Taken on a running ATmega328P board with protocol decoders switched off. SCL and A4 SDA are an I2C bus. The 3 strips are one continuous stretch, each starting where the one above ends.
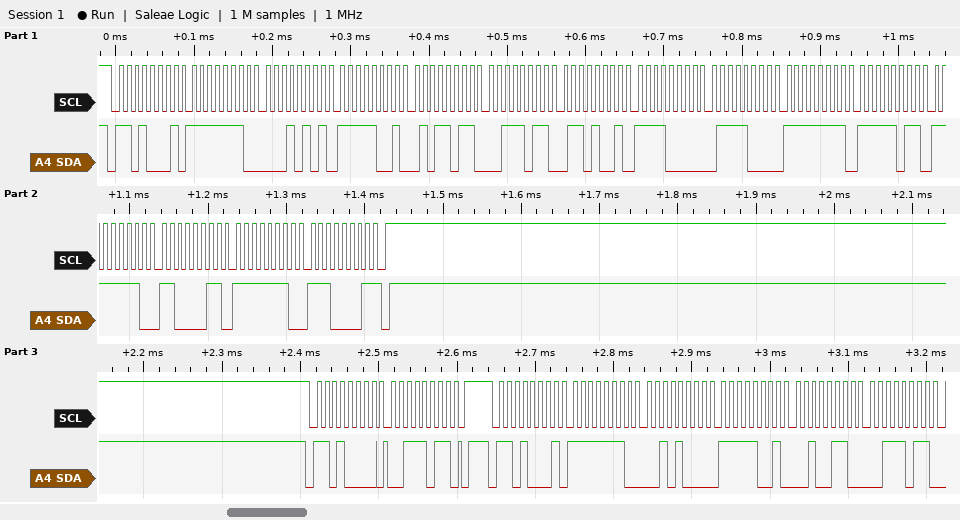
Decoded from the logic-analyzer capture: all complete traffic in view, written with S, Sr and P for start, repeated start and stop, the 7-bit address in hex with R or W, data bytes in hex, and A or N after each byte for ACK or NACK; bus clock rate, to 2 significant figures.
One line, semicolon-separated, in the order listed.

S 68R A FE A 15 A F9 A 5B A 3B A 69 A F0 A 78 A FF A FB A FE A C3 A FE A E1 N P S 68W A 3B A P S 68R A FE A 28 A F9 A 26 A 3B A; 100 kHz
